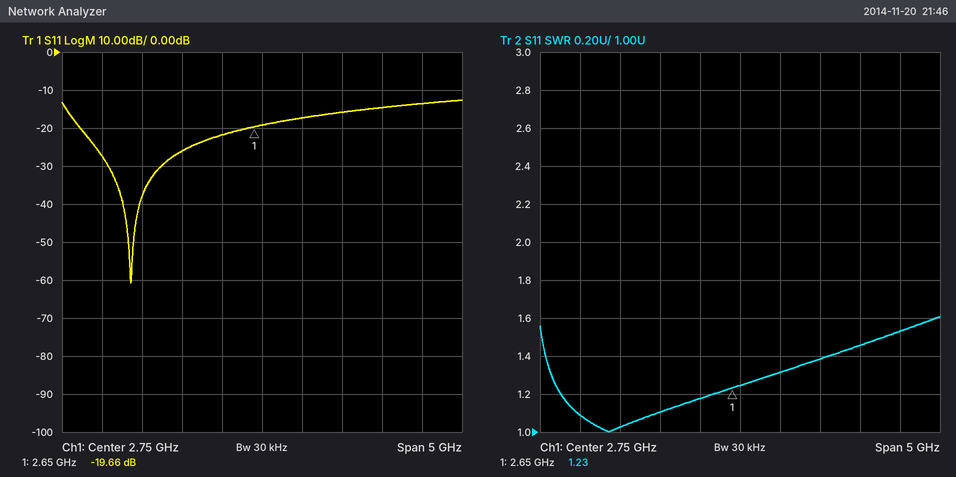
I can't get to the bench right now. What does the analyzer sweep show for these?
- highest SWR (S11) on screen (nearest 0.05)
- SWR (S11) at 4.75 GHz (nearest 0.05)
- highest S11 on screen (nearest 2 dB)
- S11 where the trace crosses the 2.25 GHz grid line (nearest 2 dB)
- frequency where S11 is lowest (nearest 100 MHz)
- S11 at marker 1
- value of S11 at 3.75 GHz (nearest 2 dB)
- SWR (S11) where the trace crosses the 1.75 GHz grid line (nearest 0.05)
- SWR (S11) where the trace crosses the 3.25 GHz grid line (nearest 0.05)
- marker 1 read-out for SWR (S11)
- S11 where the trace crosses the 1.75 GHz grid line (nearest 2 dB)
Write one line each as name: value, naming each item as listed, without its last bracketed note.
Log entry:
highest SWR (S11) on screen: 1.60
SWR (S11) at 4.75 GHz: 1.55
highest S11 on screen: -12 dB
S11 where the trace crosses the 2.25 GHz grid line: -22 dB
frequency where S11 is lowest: 1.1 GHz
S11 at marker 1: -19.66 dB
value of S11 at 3.75 GHz: -16 dB
SWR (S11) where the trace crosses the 1.75 GHz grid line: 1.10
SWR (S11) where the trace crosses the 3.25 GHz grid line: 1.30
marker 1 read-out for SWR: 1.23
S11 where the trace crosses the 1.75 GHz grid line: -26 dB
